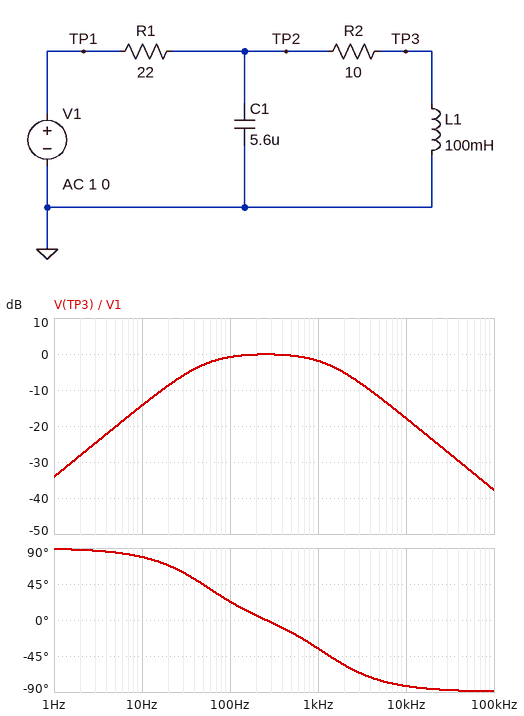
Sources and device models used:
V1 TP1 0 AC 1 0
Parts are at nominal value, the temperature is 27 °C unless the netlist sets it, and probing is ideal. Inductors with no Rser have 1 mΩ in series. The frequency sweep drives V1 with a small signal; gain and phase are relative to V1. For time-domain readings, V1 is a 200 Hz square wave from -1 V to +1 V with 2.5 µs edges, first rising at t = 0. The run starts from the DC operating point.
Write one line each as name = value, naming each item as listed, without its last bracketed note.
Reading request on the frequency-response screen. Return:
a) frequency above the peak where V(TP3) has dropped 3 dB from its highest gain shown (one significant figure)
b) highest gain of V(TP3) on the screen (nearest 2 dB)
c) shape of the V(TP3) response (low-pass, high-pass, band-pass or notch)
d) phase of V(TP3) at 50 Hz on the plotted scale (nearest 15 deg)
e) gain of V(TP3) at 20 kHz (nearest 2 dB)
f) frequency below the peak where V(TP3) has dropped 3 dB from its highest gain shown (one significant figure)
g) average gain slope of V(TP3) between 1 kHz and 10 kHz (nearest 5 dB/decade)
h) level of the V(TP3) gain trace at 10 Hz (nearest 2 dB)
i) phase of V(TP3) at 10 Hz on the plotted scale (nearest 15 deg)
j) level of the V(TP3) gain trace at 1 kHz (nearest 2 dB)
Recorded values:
frequency above the peak where V(TP3) has dropped 3 dB from its highest gain shown = 1 kHz
highest gain of V(TP3) on the screen = 0 dB
shape of the V(TP3) response = band-pass
phase of V(TP3) at 50 Hz on the plotted scale = 45 deg
gain of V(TP3) at 20 kHz = -24 dB
frequency below the peak where V(TP3) has dropped 3 dB from its highest gain shown = 50 Hz
average gain slope of V(TP3) between 1 kHz and 10 kHz = -15 dB/decade
level of the V(TP3) gain trace at 10 Hz = -14 dB
phase of V(TP3) at 10 Hz on the plotted scale = 75 deg
level of the V(TP3) gain trace at 1 kHz = -2 dB
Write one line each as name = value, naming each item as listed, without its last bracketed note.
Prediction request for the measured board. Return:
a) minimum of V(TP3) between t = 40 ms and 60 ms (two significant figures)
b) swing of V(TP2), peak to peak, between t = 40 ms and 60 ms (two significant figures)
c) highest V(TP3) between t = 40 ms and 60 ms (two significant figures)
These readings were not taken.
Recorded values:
minimum of V(TP3) between t = 40 ms and 60 ms = -1.2 V
swing of V(TP2), peak to peak, between t = 40 ms and 60 ms = 2.3 V
highest V(TP3) between t = 40 ms and 60 ms = 1.2 V
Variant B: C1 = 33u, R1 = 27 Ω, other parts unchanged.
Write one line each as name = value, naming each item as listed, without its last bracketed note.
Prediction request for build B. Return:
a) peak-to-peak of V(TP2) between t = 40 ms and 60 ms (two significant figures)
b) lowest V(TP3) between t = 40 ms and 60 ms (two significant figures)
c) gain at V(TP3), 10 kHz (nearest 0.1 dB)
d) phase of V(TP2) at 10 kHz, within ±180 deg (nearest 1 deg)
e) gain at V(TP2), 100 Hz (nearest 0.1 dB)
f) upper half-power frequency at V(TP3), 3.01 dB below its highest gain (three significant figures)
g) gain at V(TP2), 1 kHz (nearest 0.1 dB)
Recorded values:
peak-to-peak of V(TP2) between t = 40 ms and 60 ms = 1.8 V
lowest V(TP3) between t = 40 ms and 60 ms = -850 mV
gain at V(TP3), 10 kHz = -35.0 dB
phase of V(TP2) at 10 kHz, within ±180 deg = -89 deg
gain at V(TP2), 100 Hz = -0.6 dB
upper half-power frequency at V(TP3), 3.01 dB below its highest gain = 239 Hz
gain at V(TP2), 1 kHz = -15.0 dB
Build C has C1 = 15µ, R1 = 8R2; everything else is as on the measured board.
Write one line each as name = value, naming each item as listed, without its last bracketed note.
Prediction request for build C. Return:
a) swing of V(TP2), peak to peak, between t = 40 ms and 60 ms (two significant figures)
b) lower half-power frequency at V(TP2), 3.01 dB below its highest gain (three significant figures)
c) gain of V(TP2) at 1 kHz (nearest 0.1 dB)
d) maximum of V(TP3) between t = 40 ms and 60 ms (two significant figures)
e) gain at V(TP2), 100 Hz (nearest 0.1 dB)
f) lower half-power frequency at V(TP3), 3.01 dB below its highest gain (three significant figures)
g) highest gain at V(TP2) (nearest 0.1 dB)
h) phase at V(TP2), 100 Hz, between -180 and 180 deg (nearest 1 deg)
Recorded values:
swing of V(TP2), peak to peak, between t = 40 ms and 60 ms = 2.1 V
lower half-power frequency at V(TP2), 3.01 dB below its highest gain = 17.5 Hz
gain of V(TP2) at 1 kHz = -2.0 dB
maximum of V(TP3) between t = 40 ms and 60 ms = 1.1 V
gain at V(TP2), 100 Hz = -0.2 dB
lower half-power frequency at V(TP3), 3.01 dB below its highest gain = 28.0 Hz
highest gain at V(TP2) = -0.1 dB
phase at V(TP2), 100 Hz, between -180 and 180 deg = 3 deg
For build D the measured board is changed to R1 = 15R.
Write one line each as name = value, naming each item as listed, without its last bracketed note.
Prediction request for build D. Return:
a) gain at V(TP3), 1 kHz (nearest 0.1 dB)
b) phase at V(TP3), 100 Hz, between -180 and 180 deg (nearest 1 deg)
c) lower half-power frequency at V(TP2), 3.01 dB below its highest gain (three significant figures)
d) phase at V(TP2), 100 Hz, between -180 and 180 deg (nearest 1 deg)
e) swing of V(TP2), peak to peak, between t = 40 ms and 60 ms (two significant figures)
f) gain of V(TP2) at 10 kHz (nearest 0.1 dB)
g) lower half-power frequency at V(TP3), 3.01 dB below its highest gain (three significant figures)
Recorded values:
gain at V(TP3), 1 kHz = -1.0 dB
phase at V(TP3), 100 Hz, between -180 and 180 deg = 19 deg
lower half-power frequency at V(TP2), 3.01 dB below its highest gain = 31.9 Hz
phase at V(TP2), 100 Hz, between -180 and 180 deg = 10 deg
swing of V(TP2), peak to peak, between t = 40 ms and 60 ms = 2.2 V
gain of V(TP2) at 10 kHz = -14.6 dB
lower half-power frequency at V(TP3), 3.01 dB below its highest gain = 38.7 Hz
